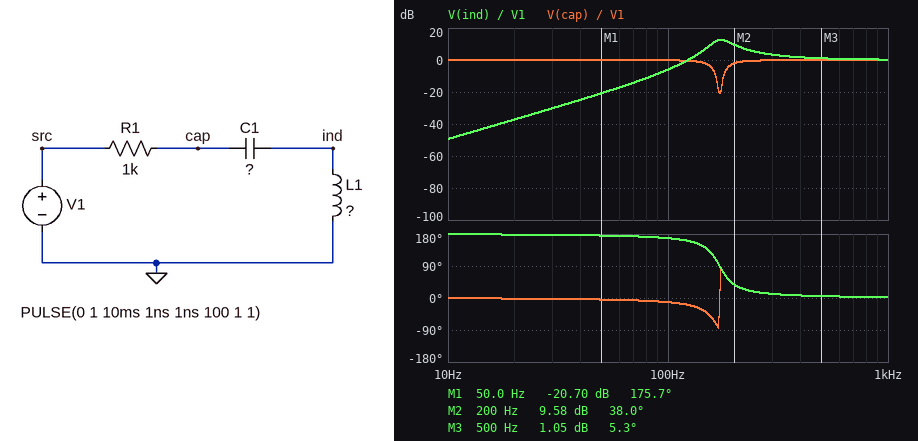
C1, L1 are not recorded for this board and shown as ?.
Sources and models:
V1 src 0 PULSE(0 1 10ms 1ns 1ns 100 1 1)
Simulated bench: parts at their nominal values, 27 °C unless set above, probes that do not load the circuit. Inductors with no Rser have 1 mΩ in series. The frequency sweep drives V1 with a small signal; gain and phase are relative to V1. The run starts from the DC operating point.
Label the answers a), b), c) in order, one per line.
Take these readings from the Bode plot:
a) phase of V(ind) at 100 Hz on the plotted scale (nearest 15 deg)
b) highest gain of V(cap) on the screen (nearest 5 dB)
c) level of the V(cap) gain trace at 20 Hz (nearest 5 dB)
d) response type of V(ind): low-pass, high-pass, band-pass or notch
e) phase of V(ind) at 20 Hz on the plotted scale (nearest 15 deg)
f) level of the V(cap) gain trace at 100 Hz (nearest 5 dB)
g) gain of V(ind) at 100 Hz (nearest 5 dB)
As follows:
a) 165 deg
b) 0 dB
c) 0 dB
d) high-pass
e) 180 deg
f) 0 dB
g) -5 dB
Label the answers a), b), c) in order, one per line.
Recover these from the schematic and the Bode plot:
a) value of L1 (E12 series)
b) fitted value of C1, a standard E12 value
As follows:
a) 3.9 H
b) 220 nF
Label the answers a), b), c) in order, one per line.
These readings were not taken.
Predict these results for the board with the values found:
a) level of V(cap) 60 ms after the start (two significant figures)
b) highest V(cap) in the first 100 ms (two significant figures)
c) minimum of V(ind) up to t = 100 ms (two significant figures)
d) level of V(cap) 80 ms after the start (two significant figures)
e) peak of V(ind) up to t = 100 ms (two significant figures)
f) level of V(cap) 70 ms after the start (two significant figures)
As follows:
a) 1.0 V
b) 1.1 V
c) -710 mV
d) 1.0 V
e) 1.0 V
f) 1.0 V
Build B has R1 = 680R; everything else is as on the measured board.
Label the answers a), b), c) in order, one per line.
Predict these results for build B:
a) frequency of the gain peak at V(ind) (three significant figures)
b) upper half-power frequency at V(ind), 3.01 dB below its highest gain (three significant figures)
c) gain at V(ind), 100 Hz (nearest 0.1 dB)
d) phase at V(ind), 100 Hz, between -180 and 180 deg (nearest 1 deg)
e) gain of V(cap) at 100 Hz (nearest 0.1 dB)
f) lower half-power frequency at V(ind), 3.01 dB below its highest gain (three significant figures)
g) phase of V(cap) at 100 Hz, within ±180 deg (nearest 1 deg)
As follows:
a) 173 Hz
b) 189 Hz
c) -5.9 dB
d) 172 deg
e) -0.1 dB
f) 160 Hz
g) -8 deg
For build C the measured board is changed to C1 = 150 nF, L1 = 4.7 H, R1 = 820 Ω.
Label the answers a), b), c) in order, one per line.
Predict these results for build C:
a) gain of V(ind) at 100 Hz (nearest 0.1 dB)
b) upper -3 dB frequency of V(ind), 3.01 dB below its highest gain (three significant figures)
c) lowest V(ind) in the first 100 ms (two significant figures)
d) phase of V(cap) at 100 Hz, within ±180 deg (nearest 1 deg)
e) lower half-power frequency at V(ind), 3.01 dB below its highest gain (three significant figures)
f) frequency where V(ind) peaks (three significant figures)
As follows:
a) -8.3 dB
b) 206 Hz
c) -800 mV
d) -6 deg
e) 178 Hz
f) 191 Hz
